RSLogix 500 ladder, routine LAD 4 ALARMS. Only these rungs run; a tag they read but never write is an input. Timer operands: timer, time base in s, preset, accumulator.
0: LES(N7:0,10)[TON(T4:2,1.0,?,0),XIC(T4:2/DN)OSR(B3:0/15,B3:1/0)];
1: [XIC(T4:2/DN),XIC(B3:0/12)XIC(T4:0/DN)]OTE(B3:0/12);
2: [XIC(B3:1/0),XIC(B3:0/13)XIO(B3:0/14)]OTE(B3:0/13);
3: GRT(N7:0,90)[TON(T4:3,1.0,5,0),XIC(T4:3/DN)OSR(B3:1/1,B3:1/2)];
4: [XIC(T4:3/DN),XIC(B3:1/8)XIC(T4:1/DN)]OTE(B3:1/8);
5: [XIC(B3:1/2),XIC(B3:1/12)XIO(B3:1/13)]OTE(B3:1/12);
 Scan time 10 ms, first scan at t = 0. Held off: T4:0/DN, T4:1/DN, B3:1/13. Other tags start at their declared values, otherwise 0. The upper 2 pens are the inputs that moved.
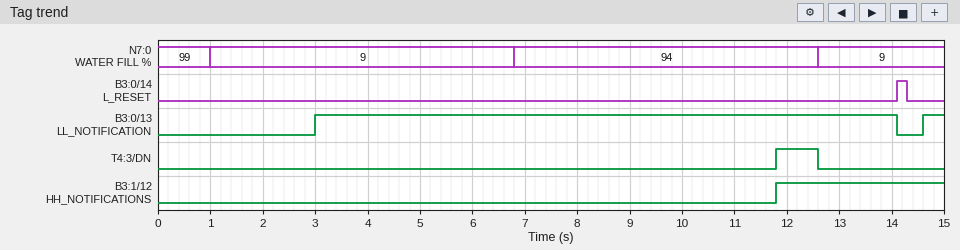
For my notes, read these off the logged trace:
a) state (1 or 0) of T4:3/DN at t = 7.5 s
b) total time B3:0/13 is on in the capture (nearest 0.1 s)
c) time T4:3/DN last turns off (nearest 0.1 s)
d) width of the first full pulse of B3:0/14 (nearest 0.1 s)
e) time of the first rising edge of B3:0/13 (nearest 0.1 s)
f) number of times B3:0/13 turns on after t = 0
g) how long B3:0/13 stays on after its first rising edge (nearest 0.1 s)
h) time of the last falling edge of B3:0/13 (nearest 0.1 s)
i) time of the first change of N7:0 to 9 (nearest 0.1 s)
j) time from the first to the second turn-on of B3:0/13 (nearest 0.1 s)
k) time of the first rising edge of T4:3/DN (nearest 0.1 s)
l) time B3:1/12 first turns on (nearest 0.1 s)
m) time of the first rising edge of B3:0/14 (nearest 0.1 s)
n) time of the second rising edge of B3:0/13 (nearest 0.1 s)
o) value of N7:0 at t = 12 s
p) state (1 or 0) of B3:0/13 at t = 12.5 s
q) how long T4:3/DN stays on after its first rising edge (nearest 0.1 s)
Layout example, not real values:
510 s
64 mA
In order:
0
11.5 s
12.6 s
0.2 s
3.0 s
2
11.1 s
14.1 s
1.0 s
11.6 s
11.8 s
11.8 s
14.1 s
14.6 s
94
1
0.8 s
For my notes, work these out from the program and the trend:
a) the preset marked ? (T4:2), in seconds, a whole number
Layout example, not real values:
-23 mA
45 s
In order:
2 s
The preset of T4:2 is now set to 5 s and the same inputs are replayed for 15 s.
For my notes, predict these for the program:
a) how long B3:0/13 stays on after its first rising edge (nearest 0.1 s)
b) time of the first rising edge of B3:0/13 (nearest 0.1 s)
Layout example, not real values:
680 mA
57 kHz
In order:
8.1 s
6.0 s
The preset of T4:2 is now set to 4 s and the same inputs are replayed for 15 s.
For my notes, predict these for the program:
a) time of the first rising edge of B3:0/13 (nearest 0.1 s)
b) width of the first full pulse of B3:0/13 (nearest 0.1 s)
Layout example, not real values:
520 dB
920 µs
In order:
5.0 s
9.1 s
